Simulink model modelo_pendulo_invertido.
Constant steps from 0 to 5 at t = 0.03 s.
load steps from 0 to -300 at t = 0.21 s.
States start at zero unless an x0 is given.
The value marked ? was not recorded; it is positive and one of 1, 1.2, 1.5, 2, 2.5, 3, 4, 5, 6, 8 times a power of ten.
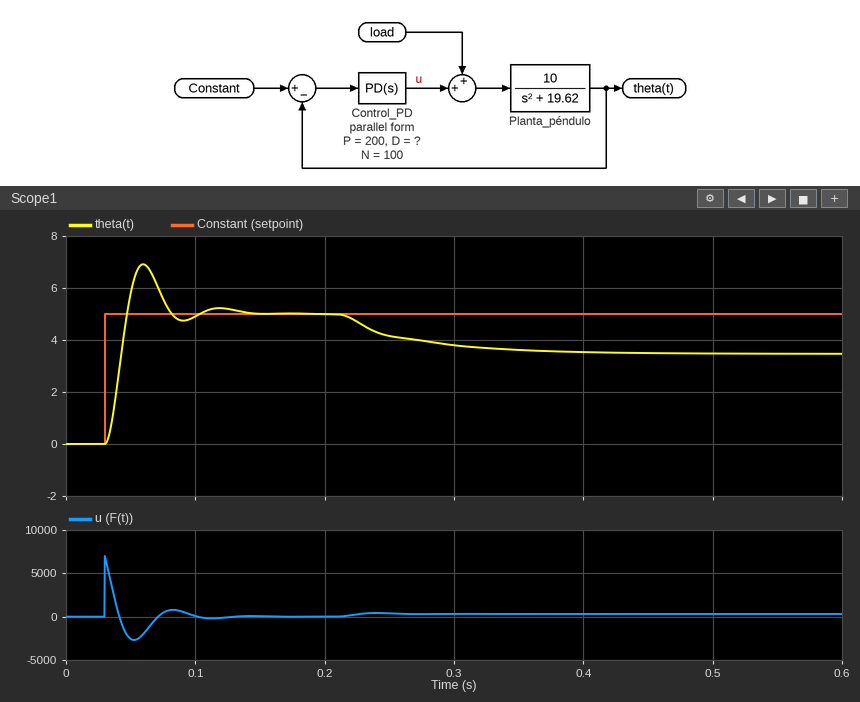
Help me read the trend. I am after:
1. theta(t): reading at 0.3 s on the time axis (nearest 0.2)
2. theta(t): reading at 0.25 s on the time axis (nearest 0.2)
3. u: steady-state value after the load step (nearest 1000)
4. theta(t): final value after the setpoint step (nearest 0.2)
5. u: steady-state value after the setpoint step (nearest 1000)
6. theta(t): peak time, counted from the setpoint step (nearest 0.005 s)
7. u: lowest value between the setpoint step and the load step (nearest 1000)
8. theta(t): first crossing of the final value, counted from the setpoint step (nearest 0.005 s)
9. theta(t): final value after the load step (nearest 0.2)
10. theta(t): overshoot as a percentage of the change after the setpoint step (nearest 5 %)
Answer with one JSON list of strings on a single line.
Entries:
["3.8", "4.2", "0", "5.0", "0", "0.030 s", "-3000", "0.015 s", "3.4", "40 %"]
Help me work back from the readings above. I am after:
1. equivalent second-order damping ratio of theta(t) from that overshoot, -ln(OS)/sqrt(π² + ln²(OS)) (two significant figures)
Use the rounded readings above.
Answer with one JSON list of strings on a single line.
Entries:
["0.28"]
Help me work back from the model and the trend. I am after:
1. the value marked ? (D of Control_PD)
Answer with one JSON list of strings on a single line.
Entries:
["12"]
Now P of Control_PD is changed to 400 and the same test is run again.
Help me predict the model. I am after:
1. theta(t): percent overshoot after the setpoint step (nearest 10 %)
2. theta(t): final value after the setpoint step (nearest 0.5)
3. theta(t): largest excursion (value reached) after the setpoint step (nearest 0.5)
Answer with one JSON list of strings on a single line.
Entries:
["50 %", "5.0", "7.5"]
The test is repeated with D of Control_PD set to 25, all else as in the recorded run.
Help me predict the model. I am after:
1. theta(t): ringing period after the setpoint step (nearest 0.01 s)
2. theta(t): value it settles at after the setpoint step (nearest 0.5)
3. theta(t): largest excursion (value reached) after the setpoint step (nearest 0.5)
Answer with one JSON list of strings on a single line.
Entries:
["0.04 s", "5.0", "7.0"]
